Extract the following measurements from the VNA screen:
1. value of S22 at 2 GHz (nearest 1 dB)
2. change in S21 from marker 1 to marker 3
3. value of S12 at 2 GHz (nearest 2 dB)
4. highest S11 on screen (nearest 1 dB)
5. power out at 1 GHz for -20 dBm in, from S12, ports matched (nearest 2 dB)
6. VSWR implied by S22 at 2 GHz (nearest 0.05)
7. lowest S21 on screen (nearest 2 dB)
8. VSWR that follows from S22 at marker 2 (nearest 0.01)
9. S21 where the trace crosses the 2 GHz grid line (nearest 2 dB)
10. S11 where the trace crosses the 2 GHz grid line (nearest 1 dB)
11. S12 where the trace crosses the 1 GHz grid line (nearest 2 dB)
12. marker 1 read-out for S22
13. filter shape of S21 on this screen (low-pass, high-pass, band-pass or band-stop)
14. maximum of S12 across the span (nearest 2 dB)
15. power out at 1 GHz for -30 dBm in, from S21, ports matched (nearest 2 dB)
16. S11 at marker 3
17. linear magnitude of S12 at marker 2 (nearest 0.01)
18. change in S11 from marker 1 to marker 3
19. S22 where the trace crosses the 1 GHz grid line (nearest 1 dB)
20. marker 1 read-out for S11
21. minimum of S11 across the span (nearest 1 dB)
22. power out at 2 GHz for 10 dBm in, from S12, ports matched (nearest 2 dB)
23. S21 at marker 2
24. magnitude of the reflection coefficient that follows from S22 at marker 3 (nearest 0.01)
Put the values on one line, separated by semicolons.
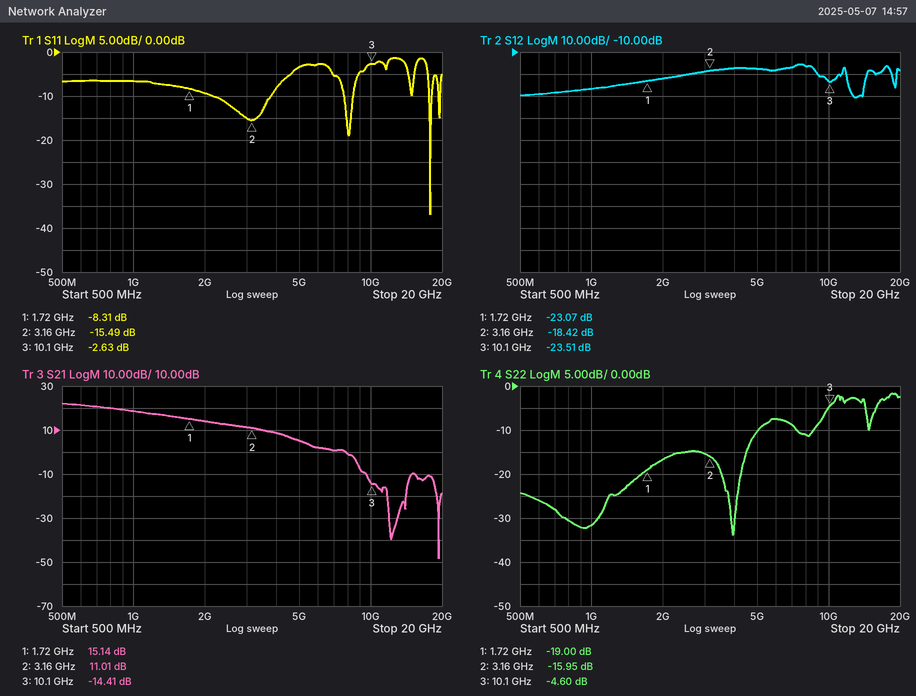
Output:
-17 dB; -29.55 dB; -22 dB; -1 dB; -46 dBm; 1.35; -48 dB; 1.38; 14 dB; -9 dB; -26 dB; -19.00 dB; low-pass; -16 dB; -12 dBm; -2.63 dB; 0.12; 5.68 dB; -32 dB; -8.31 dB; -37 dB; -12 dBm; 11.01 dB; 0.59
